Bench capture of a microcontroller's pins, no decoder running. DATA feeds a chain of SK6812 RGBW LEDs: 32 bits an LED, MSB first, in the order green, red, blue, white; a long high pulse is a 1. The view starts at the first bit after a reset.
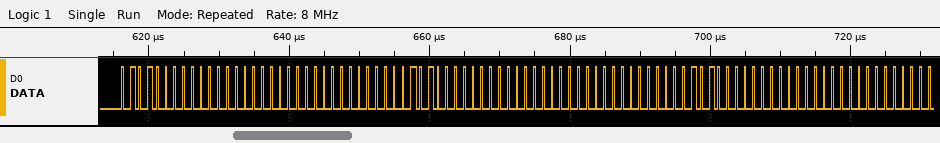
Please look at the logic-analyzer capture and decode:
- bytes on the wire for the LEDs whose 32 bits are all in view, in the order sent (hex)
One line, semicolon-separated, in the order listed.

50 00 00 00 50 00 00 00
